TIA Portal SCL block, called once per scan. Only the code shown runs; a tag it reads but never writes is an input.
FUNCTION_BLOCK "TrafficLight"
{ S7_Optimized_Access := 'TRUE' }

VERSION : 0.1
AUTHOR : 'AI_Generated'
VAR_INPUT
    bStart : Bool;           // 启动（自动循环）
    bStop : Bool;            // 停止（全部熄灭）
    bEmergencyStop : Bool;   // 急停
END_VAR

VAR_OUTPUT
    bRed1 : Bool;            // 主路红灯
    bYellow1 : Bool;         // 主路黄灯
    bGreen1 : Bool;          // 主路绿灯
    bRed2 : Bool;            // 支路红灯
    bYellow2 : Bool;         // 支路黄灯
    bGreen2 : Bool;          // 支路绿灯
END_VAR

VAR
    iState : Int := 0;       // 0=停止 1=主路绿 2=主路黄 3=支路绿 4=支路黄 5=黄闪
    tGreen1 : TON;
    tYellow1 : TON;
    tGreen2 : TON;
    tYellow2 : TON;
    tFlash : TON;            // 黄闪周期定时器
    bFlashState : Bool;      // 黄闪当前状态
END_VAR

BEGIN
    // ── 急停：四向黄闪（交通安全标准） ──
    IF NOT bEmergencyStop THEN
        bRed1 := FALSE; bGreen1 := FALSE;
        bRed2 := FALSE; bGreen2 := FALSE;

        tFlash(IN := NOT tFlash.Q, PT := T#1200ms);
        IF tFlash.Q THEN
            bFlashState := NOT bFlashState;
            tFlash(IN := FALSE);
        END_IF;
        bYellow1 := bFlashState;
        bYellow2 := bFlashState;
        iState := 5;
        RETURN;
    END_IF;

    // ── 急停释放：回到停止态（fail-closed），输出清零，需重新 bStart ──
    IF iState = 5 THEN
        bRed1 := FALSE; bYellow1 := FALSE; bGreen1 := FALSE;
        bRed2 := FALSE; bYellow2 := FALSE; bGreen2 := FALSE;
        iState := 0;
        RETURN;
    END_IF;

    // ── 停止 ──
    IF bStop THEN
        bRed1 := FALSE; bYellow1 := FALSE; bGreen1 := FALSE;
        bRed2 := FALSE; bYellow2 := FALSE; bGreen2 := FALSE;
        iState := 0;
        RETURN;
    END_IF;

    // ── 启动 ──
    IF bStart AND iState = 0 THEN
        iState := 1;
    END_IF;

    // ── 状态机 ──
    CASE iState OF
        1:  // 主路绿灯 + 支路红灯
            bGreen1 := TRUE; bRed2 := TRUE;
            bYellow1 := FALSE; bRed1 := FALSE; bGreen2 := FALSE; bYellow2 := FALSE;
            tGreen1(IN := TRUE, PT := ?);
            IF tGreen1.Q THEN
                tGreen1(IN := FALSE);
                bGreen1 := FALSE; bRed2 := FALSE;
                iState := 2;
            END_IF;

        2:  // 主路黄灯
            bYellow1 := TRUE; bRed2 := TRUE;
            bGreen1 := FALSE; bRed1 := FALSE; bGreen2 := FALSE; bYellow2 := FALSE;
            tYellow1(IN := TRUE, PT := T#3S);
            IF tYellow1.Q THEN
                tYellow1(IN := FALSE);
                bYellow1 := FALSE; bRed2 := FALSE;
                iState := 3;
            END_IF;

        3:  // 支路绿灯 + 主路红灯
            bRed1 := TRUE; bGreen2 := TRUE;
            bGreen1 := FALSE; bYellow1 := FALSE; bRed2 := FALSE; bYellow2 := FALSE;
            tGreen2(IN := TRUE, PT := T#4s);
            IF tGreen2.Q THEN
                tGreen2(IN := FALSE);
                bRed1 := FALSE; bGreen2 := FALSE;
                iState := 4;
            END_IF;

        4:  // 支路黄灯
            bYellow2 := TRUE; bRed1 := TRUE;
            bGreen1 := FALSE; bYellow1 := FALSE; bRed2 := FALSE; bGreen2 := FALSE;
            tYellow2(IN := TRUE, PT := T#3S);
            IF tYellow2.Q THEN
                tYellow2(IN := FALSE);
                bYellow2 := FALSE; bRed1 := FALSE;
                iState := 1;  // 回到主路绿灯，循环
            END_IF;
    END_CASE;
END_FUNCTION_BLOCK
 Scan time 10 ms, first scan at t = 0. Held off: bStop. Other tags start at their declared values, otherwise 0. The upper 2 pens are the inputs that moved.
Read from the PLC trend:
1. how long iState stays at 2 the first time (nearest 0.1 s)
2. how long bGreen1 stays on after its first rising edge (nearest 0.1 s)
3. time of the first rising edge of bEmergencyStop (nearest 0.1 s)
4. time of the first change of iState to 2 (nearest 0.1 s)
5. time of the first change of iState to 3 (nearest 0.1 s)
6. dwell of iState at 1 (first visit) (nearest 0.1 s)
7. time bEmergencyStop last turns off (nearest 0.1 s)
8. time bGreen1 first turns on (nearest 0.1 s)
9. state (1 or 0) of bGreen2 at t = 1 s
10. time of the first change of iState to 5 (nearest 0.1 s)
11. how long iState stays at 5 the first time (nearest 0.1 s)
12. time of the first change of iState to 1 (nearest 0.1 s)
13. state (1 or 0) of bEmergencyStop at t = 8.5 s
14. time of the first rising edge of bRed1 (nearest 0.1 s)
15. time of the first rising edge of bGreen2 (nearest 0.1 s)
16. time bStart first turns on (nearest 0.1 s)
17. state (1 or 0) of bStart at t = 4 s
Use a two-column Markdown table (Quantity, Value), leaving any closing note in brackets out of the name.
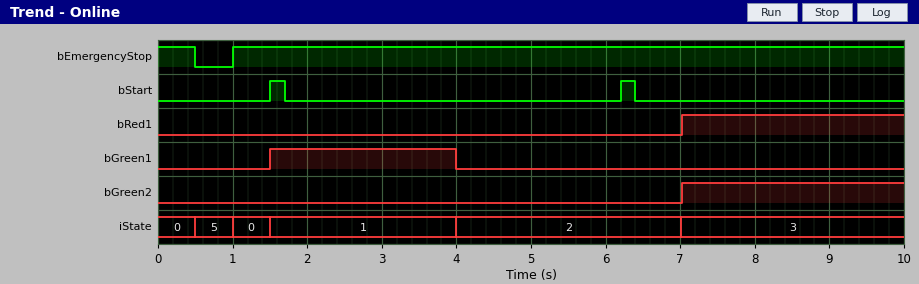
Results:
| Quantity | Value |
|---|---|
| how long iState stays at 2 the first time | 3.0 s |
| how long bGreen1 stays on after its first rising edge | 2.5 s |
| time of the first rising edge of bEmergencyStop | 1.0 s |
| time of the first change of iState to 2 | 4.0 s |
| time of the first change of iState to 3 | 7.0 s |
| dwell of iState at 1 (first visit) | 2.5 s |
| time bEmergencyStop last turns off | 0.5 s |
| time bGreen1 first turns on | 1.5 s |
| state (1 or 0) of bGreen2 at t = 1 s | 0 |
| time of the first change of iState to 5 | 0.5 s |
| how long iState stays at 5 the first time | 0.5 s |
| time of the first change of iState to 1 | 1.5 s |
| state (1 or 0) of bEmergencyStop at t = 8.5 s | 1 |
| time of the first rising edge of bRed1 | 7.0 s |
| time of the first rising edge of bGreen2 | 7.0 s |
| time bStart first turns on | 1.5 s |
| state (1 or 0) of bStart at t = 4 s | 0 |
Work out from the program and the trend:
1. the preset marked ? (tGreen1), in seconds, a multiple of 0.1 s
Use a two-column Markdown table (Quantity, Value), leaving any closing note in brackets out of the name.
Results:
| Quantity | Value |
|---|---|
| the preset marked ? (tGreen1), in seconds, a multiple of 0.1 s | 2.5 s |
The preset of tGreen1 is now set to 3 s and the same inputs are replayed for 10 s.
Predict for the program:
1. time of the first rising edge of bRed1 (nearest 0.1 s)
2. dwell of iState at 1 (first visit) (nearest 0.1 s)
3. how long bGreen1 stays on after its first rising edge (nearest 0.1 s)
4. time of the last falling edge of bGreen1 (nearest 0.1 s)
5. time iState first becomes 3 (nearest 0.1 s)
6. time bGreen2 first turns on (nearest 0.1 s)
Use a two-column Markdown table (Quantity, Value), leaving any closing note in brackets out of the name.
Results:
| Quantity | Value |
|---|---|
| time of the first rising edge of bRed1 | 7.5 s |
| dwell of iState at 1 (first visit) | 3.0 s |
| how long bGreen1 stays on after its first rising edge | 3.0 s |
| time of the last falling edge of bGreen1 | 4.5 s |
| time iState first becomes 3 | 7.5 s |
| time bGreen2 first turns on | 7.5 s |
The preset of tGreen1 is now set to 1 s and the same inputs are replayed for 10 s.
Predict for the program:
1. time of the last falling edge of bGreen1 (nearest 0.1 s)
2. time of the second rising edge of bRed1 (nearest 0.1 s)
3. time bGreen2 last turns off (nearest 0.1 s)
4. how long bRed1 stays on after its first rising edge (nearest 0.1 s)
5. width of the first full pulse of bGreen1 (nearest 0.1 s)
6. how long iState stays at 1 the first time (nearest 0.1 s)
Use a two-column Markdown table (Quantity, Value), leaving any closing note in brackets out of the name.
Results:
| Quantity | Value |
|---|---|
| time of the last falling edge of bGreen1 | 2.5 s |
| time of the second rising edge of bRed1 | 9.5 s |
| time bGreen2 last turns off | 9.5 s |
| how long bRed1 stays on after its first rising edge | 4.0 s |
| width of the first full pulse of bGreen1 | 1.0 s |
| how long iState stays at 1 the first time | 1.0 s |
